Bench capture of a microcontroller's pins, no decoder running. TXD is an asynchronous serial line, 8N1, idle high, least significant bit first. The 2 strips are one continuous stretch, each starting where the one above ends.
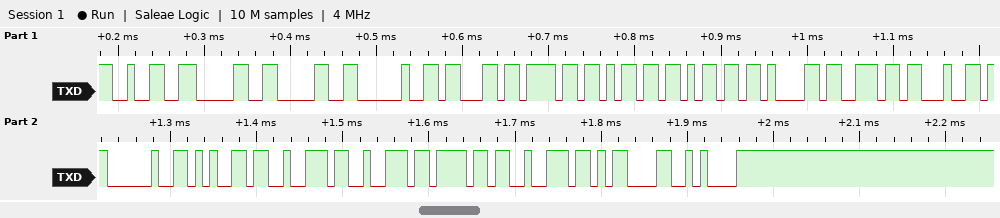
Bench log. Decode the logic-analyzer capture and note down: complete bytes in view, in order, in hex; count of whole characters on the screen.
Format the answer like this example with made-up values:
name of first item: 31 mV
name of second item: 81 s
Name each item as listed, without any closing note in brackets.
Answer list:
complete bytes in view, in order, in hex: 32 30 30 20 63 6F 6D 6D 61 6E 64 20 65 72 72 6F 72 0D 0A
count of whole characters on the screen: 19
